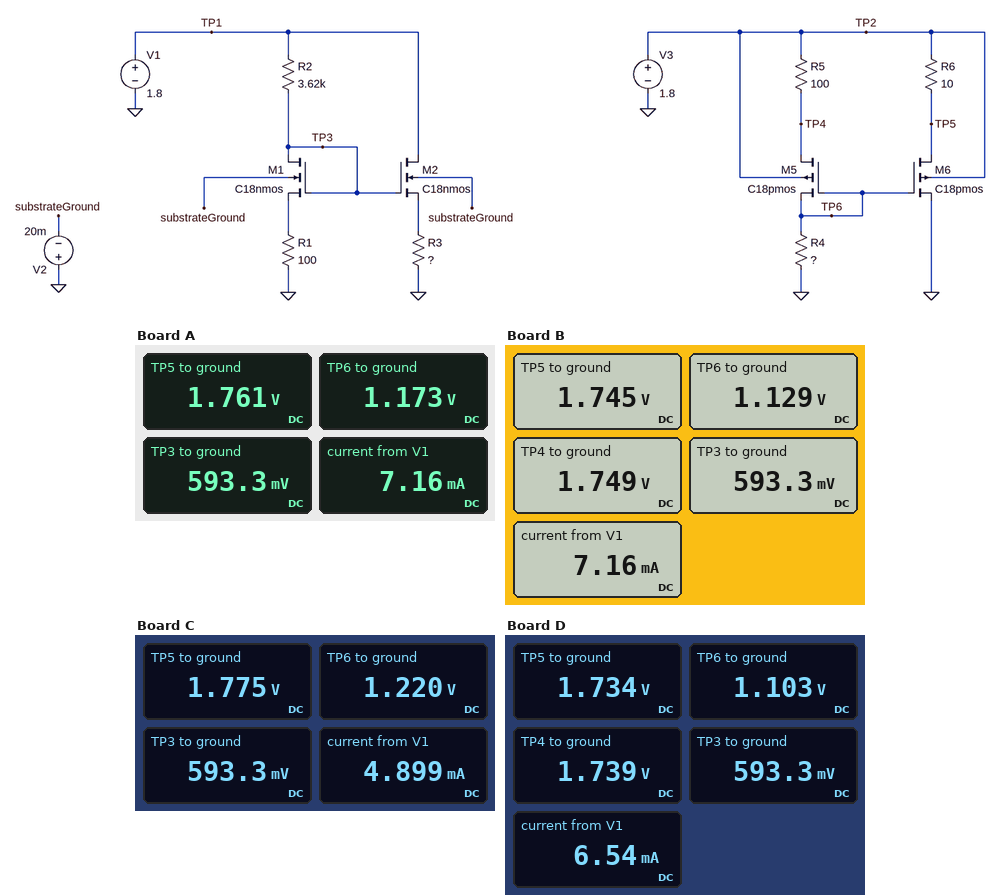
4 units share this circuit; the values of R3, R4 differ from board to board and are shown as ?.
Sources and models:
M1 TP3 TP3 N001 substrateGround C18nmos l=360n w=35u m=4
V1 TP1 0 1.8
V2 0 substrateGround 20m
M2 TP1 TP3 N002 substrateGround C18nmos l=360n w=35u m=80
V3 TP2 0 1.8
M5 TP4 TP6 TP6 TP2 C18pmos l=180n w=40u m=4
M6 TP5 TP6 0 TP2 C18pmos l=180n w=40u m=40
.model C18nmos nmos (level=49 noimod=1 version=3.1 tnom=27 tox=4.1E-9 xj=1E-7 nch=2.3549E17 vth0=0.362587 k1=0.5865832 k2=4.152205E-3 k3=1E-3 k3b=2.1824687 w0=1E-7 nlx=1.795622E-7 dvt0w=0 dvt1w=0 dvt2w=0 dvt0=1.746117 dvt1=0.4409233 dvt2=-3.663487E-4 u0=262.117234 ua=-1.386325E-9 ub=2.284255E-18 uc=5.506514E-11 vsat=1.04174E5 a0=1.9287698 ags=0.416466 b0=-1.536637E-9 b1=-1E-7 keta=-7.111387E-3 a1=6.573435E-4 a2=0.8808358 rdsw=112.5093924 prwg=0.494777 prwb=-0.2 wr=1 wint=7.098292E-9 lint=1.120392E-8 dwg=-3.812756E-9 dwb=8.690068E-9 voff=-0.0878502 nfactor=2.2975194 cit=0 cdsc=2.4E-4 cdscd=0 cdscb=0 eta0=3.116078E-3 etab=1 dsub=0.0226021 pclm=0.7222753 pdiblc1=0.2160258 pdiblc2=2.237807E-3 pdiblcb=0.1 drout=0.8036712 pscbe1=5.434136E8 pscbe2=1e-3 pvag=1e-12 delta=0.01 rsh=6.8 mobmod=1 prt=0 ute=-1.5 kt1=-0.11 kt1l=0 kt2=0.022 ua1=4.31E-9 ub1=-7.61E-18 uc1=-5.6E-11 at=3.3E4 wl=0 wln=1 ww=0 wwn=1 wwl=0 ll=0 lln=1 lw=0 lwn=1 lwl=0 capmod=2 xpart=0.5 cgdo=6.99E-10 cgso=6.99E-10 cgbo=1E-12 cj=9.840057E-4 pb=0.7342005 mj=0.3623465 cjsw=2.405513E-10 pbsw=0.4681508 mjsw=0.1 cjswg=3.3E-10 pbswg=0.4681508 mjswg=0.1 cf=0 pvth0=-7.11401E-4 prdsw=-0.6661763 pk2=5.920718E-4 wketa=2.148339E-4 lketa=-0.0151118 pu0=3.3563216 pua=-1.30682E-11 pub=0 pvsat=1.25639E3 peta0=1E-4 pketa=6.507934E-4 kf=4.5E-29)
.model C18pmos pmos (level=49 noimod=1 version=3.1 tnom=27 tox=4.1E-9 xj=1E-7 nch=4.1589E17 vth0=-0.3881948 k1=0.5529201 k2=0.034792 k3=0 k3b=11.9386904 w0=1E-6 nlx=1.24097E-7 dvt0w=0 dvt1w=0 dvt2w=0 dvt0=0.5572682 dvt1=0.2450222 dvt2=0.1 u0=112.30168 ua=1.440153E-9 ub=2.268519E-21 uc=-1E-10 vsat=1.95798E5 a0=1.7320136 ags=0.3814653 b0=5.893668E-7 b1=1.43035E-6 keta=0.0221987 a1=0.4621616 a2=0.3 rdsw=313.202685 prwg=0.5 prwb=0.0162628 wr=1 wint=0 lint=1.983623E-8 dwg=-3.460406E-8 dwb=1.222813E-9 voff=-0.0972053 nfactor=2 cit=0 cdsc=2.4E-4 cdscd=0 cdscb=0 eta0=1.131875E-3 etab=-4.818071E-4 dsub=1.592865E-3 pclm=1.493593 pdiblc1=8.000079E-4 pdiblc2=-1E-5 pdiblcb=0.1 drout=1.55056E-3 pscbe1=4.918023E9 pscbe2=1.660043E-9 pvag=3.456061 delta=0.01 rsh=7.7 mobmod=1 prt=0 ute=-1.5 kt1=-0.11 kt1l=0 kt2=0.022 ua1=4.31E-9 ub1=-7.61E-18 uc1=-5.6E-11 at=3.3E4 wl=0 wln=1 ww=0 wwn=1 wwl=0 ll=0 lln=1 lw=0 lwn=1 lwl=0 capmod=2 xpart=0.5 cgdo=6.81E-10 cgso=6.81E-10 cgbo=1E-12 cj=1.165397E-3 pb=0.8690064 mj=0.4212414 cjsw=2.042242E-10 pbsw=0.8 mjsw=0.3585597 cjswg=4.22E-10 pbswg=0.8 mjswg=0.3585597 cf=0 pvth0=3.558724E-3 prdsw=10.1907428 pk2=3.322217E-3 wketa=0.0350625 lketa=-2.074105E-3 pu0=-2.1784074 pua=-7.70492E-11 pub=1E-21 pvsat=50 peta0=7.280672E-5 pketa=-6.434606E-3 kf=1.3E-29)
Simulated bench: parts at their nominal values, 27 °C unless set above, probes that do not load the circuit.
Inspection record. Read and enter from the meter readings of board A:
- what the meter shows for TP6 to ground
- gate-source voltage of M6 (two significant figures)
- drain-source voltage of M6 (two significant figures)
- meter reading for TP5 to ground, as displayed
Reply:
1.173 V
1.2 V
1.8 V
1.761 V
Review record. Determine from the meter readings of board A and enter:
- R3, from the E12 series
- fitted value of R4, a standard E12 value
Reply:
5.6 Ω
3.3 kΩ
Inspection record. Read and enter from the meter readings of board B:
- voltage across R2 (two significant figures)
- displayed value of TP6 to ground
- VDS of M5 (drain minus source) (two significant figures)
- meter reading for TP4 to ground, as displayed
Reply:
1.2 V
1.129 V
620 mV
1.749 V
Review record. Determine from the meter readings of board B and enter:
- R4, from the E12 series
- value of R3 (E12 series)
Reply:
2.2 kΩ
5.6 Ω
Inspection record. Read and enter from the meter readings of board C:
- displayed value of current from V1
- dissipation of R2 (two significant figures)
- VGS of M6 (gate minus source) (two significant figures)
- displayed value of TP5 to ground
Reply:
4.899 mA
400 µW
1.2 V
1.775 V
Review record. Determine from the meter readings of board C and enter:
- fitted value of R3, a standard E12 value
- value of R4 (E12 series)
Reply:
12 Ω
5.6 kΩ
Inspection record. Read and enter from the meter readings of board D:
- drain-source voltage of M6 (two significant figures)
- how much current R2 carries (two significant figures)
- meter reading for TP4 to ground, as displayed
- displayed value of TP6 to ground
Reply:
1.7 V
330 µA
1.739 V
1.103 V
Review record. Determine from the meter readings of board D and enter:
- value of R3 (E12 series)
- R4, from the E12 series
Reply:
6.8 Ω
1.8 kΩ
